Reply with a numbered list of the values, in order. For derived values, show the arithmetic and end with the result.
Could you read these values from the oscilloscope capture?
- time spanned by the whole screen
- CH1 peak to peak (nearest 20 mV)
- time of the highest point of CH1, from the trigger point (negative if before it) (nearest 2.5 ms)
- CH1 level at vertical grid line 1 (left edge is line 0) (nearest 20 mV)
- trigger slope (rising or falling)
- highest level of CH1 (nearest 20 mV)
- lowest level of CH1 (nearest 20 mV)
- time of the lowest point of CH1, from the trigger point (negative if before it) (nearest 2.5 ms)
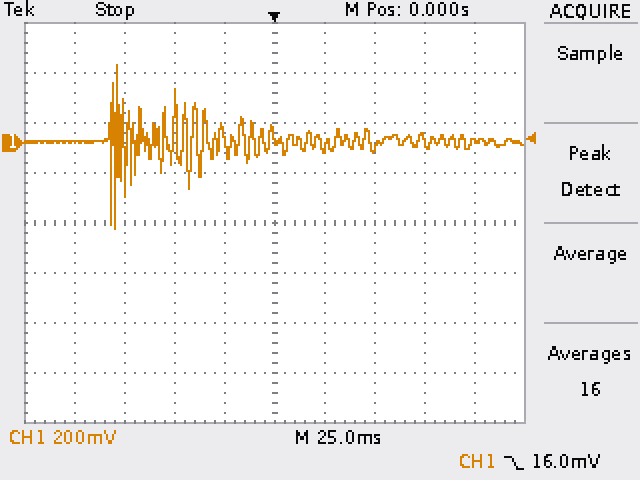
1. 250 ms
2. 320 mV − (-340 mV) = 660 mV
3. -77.5 ms
4. 0 mV
5. falling
6. 320 mV
7. -340 mV
8. -80.0 ms
